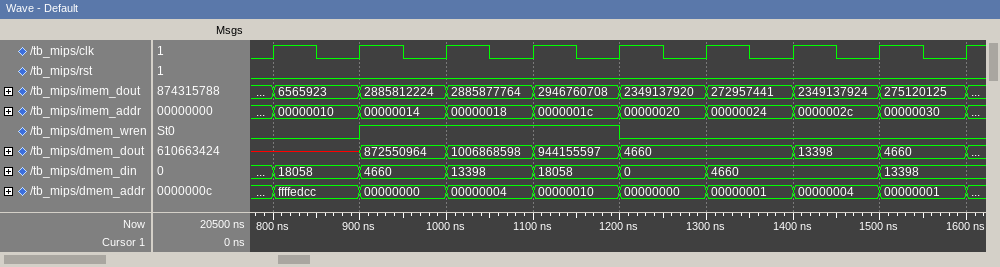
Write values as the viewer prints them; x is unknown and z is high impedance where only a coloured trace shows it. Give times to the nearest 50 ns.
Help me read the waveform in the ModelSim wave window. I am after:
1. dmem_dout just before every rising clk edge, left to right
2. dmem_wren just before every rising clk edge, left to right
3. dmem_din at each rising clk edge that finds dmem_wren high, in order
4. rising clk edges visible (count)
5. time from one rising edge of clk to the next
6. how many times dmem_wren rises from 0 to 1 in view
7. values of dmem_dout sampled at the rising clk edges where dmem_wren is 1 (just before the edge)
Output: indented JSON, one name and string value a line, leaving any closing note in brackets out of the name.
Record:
{
  "dmem_dout just before every rising clk edge, left to right": "x, x, 872550964, 1006868598, 944155597, 4660, 4660, 13398, 4660",
  "dmem_wren just before every rising clk edge, left to right": "0 0 1 1 1 0 0 0 0",
  "dmem_din at each rising clk edge that finds dmem_wren high, in order": "4660, 13398, 18058",
  "rising clk edges visible": "9",
  "time from one rising edge of clk to the next": "100 ns",
  "how many times dmem_wren rises from 0 to 1 in view": "1",
  "values of dmem_dout sampled at the rising clk edges where dmem_wren is 1": "872550964, 1006868598, 944155597"
}
